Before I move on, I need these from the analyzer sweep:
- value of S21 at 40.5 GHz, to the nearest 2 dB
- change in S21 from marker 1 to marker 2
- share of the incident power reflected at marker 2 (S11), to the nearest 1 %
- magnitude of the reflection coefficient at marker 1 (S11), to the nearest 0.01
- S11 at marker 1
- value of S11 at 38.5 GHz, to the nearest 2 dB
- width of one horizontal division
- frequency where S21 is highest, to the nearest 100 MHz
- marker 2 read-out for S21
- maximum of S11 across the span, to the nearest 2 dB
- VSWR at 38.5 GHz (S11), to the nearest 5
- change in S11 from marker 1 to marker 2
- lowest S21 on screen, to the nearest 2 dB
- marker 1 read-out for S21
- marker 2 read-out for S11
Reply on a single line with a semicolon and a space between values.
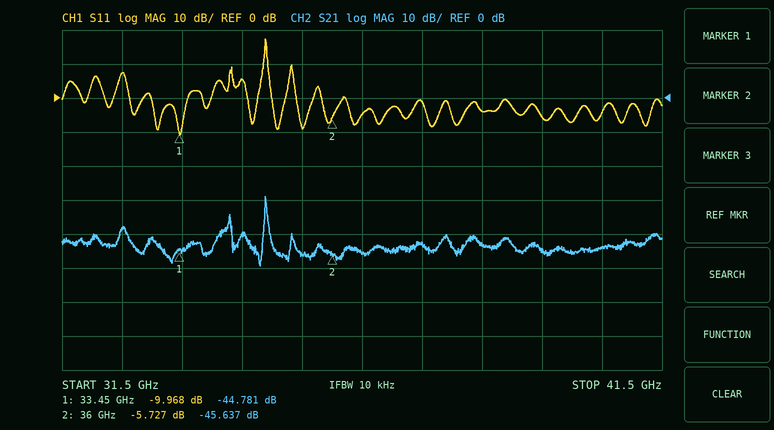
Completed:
-44 dB; -0.856 dB; 27 %; 0.32; -9.968 dB; -4 dB; 1 GHz; 34.9 GHz; -45.637 dB; 18 dB; 5; 4.241 dB; -50 dB; -44.781 dB; -5.727 dB
